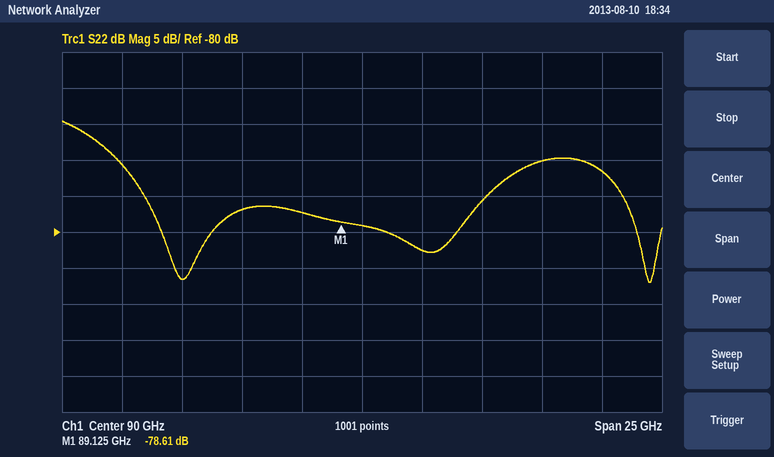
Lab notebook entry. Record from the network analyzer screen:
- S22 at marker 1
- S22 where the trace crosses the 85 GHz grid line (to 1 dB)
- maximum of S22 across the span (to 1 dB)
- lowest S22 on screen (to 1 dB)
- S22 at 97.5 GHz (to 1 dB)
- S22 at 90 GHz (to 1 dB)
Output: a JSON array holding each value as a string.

["-78.61 dB", "-77 dB", "-65 dB", "-87 dB", "-70 dB", "-79 dB"]
